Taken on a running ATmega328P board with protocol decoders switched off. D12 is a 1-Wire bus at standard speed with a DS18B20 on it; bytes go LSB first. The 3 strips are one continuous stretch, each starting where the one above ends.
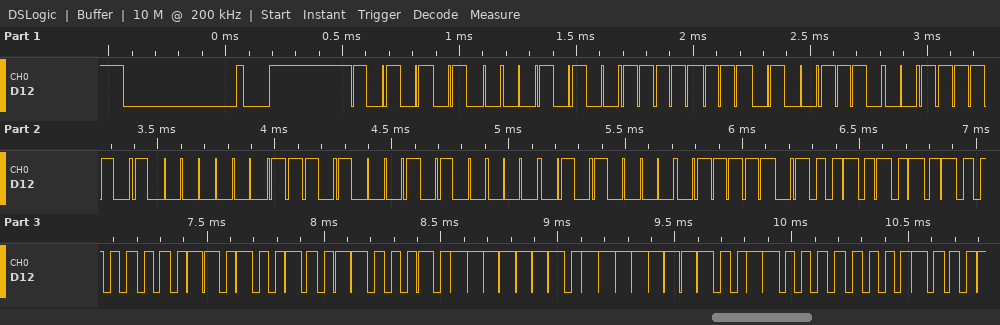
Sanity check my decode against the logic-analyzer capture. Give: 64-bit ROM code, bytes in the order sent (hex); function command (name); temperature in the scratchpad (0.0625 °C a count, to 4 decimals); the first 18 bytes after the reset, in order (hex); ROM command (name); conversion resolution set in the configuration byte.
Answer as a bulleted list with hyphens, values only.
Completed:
- 28 FF 72 7C 01 17 05 0A
- Read Scratchpad
- 21.2500 °C
- 55 28 FF 72 7C 01 17 05 0A BE 54 01 4B 46 7F FF 0C 10
- Match ROM
- 12 bits
